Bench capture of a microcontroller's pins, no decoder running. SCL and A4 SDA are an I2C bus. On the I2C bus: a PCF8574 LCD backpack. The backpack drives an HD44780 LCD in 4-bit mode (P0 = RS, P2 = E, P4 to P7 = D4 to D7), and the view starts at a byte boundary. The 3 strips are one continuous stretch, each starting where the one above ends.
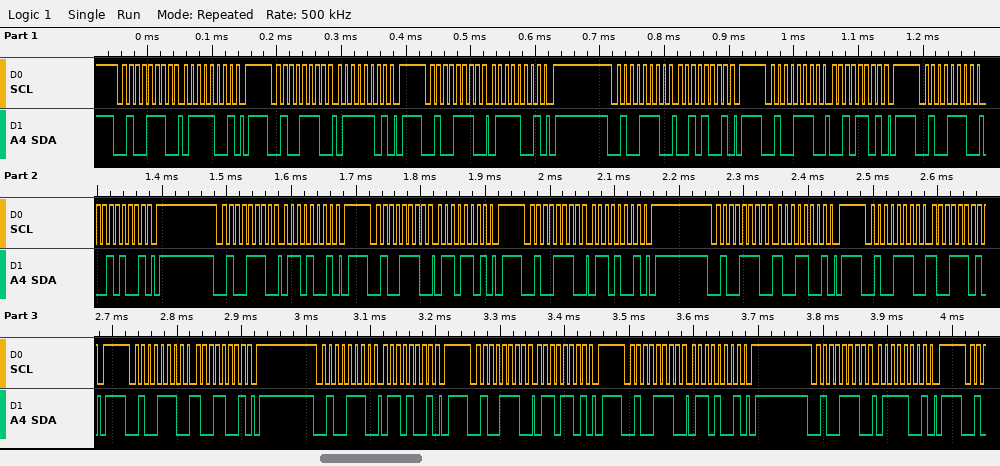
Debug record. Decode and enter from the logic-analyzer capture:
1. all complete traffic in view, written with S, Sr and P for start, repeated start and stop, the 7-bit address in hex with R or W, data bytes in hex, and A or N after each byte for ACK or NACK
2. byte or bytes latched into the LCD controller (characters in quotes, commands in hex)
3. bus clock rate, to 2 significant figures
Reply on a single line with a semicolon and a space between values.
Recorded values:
S 27W A 79 A P S 27W A 7D A P S 27W A 79 A P S 27W A 29 A P S 27W A 2D A P S 27W A 29 A P S 27W A 69 A P S 27W A 6D A P S 27W A 69 A P S 27W A 99 A P S 27W A 9D A P S 27W A 99 A P S 27W A 69 A P S 27W A 6D A P S 27W A 69 A P S 27W A 79 A P; 'r' 'i'; 100 kHz
